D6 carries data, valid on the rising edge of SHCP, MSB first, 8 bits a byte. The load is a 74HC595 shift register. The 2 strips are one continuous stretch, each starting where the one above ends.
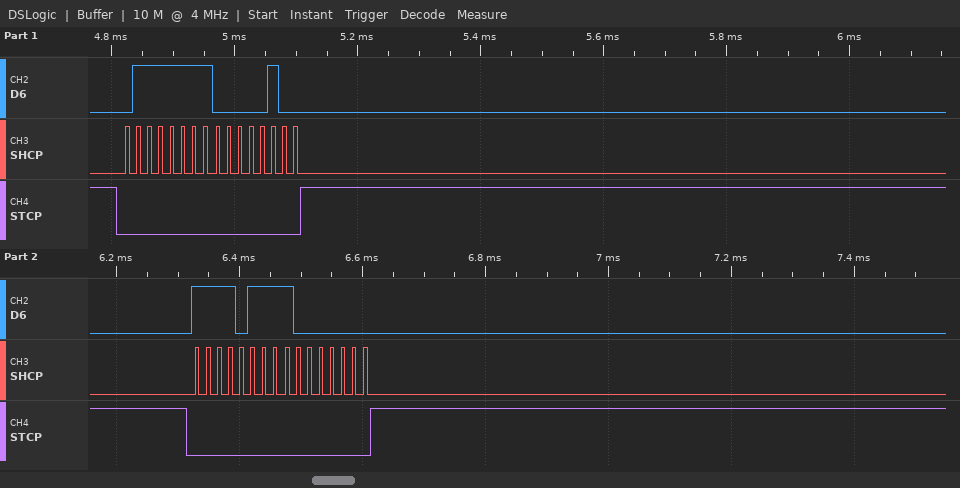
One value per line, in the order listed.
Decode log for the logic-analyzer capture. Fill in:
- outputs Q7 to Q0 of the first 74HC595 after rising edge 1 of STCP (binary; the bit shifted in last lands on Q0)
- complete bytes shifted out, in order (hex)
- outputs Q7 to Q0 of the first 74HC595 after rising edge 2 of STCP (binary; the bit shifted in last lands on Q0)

00000100
7F 04 F7 80
10000000
